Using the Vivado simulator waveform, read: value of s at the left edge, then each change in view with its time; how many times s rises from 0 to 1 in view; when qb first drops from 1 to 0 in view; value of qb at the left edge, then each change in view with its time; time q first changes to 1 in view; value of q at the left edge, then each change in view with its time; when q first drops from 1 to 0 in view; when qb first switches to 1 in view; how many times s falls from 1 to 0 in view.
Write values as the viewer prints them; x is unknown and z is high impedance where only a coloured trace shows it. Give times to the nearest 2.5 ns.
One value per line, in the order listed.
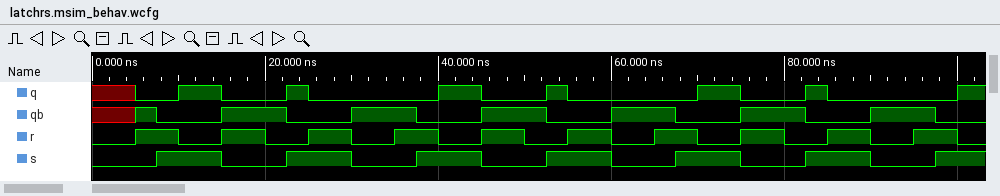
0, 1 at 7.5 ns, 0 at 15 ns, 1 at 22.5 ns, 0 at 30 ns, 1 at 37.5 ns, 0 at 45 ns, 1 at 52.5 ns, 0 at 60 ns, 1 at 67.5 ns, 0 at 75 ns, 1 at 82.5 ns, 0 at 90 ns, 1 at 97.5 ns
7
7.5 ns
x, 1 at 5 ns, 0 at 7.5 ns, 1 at 15 ns, 0 at 22.5 ns, 1 at 30 ns, 0 at 37.5 ns, 1 at 45 ns, 0 at 52.5 ns, 1 at 60 ns, 0 at 67.5 ns, 1 at 75 ns, 0 at 82.5 ns, 1 at 90 ns, 0 at 97.5 ns
10 ns
x, 0 at 5 ns, 1 at 10 ns, 0 at 15 ns, 1 at 22.5 ns, 0 at 25 ns, 1 at 40 ns, 0 at 45 ns, 1 at 52.5 ns, 0 at 55 ns, 1 at 70 ns, 0 at 75 ns, 1 at 82.5 ns, 0 at 85 ns, 1 at 100 ns
15 ns
5 ns
6
